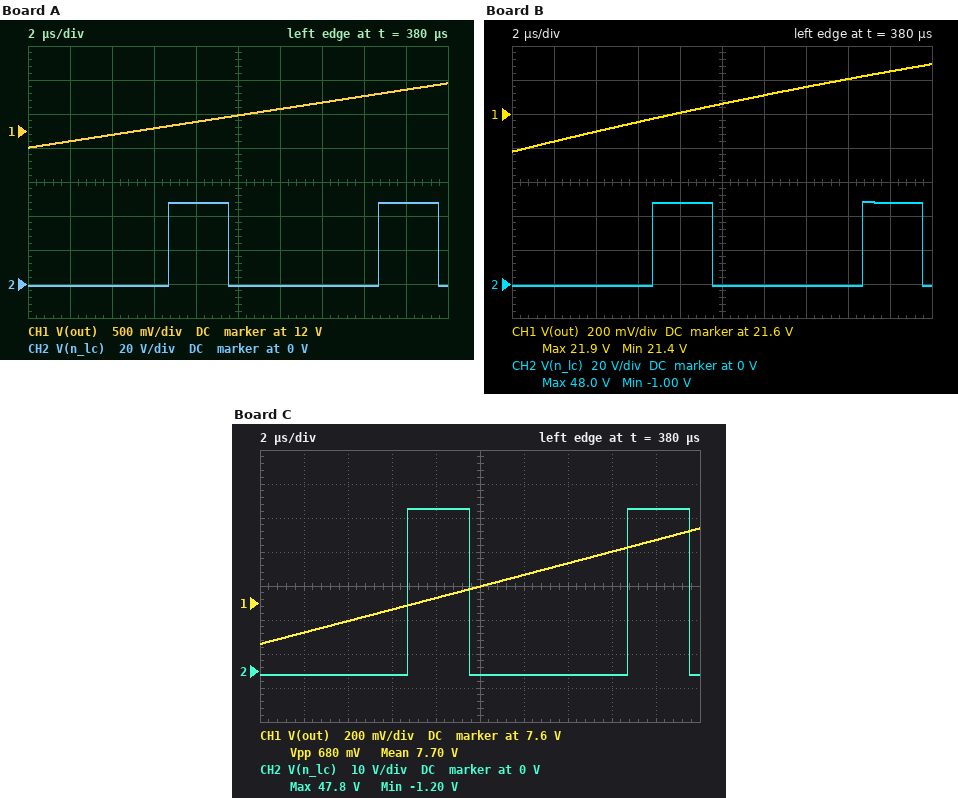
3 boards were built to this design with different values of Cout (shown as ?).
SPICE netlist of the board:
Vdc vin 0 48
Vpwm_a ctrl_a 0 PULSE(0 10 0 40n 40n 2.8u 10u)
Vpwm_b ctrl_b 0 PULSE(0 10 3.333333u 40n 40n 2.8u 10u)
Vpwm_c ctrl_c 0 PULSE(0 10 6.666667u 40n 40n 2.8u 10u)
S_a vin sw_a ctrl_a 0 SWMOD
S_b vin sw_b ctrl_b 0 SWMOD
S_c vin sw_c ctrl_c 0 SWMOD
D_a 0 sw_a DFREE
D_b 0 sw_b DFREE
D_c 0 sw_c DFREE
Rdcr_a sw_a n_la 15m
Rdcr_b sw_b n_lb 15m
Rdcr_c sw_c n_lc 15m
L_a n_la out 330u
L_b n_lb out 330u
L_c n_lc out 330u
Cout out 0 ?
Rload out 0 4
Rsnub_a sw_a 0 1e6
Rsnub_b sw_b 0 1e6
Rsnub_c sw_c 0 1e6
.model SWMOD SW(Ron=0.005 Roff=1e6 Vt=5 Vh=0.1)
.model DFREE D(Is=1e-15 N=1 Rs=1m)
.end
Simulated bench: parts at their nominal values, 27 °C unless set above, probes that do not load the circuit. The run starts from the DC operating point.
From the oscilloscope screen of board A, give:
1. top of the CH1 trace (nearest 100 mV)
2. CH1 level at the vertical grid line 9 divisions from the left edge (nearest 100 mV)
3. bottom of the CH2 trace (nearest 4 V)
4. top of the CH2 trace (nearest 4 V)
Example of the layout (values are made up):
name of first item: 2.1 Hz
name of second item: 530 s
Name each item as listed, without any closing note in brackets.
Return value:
top of the CH1 trace: 12.7 V
CH1 level at the vertical grid line 9 divisions from the left edge: 12.6 V
bottom of the CH2 trace: 0 V
top of the CH2 trace: 48 V
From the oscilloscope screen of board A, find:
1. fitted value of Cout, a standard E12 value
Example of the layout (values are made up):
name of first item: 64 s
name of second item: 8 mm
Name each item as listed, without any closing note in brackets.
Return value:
fitted value of Cout, a standard E12 value: 560 µF
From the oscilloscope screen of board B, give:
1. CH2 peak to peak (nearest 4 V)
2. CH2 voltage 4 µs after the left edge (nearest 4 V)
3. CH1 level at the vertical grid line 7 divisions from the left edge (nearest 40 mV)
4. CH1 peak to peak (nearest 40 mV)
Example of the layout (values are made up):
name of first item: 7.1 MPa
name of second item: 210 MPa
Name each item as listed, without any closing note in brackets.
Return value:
CH2 peak to peak: 48 V
CH2 voltage 4 µs after the left edge: 0 V
CH1 level at the vertical grid line 7 divisions from the left edge: 21.76 V
CH1 peak to peak: 520 mV
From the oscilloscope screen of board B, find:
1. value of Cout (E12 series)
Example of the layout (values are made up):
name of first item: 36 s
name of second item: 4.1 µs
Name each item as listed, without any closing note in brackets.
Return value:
value of Cout: 180 µF
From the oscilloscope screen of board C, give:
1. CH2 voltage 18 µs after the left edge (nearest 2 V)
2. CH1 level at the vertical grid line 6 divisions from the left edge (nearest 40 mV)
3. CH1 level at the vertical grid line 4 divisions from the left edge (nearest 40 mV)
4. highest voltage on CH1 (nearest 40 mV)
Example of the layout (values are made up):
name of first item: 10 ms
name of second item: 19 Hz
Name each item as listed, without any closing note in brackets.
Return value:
CH2 voltage 18 µs after the left edge: 48 V
CH1 level at the vertical grid line 6 divisions from the left edge: 7.76 V
CH1 level at the vertical grid line 4 divisions from the left edge: 7.64 V
highest voltage on CH1: 8.04 V
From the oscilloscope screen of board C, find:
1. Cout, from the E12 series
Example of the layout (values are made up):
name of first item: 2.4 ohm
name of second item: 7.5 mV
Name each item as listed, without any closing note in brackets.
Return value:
Cout, from the E12 series: 1 mF
